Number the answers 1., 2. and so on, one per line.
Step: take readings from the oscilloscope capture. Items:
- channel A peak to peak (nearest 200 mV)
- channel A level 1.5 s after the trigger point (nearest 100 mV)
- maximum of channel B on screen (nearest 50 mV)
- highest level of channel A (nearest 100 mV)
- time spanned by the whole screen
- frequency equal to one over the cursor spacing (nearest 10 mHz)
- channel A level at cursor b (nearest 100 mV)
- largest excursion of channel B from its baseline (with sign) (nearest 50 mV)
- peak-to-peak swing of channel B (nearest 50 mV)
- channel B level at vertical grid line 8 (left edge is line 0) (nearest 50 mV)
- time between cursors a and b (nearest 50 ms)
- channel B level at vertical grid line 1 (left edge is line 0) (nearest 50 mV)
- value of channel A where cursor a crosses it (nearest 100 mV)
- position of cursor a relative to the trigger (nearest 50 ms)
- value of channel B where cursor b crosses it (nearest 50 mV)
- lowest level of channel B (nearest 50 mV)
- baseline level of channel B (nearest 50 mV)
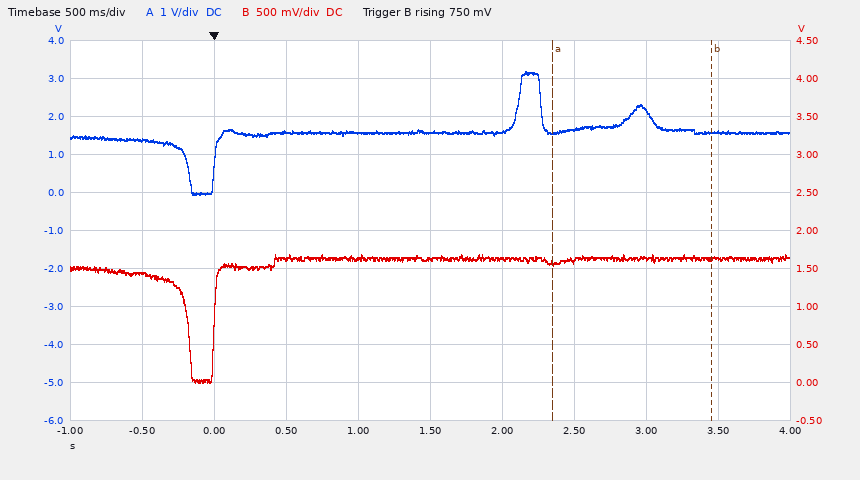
1. 3.2 V
2. 1.6 V
3. 1.70 V
4. 3.2 V
5. 5 s
6. 910 mHz
7. 1.6 V
8. -1.65 V
9. 1.70 V
10. 1.65 V
11. 1.10 s
12. 1.45 V
13. 1.6 V
14. +2.35 s
15. 1.65 V
16. 0 mV
17. 1.65 V
